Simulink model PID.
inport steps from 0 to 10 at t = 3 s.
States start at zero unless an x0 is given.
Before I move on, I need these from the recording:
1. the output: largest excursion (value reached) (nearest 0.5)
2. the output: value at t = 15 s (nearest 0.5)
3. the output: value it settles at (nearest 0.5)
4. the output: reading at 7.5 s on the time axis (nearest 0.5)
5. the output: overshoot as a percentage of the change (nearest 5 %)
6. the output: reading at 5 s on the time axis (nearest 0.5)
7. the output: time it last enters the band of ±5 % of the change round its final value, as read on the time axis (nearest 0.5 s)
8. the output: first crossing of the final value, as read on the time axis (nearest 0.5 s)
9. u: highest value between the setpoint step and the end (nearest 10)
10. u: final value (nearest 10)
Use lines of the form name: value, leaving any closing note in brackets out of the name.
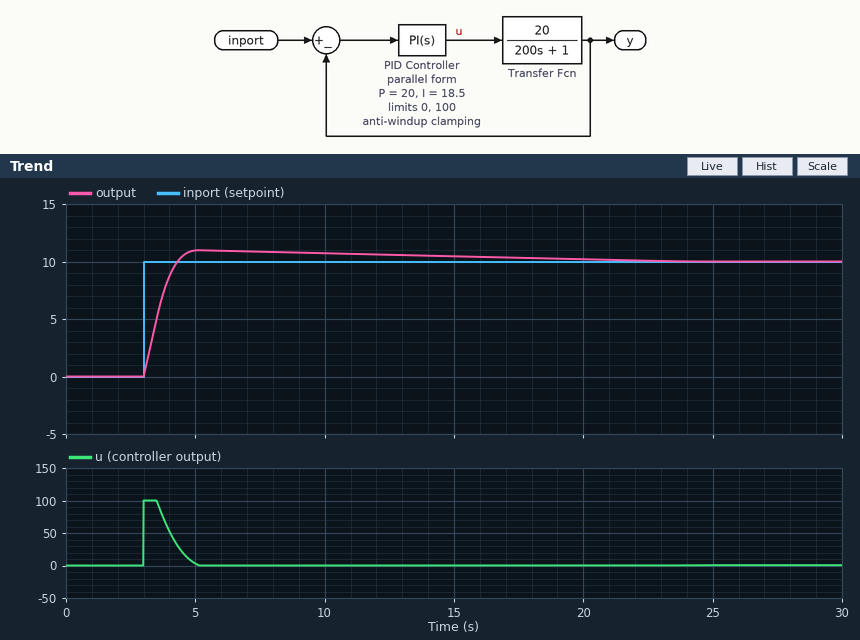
the output: largest excursion (value reached): 11.0
the output: value at t = 15 s: 10.5
the output: value it settles at: 10.0
the output: reading at 7.5 s on the time axis: 11.0
the output: overshoot as a percentage of the change: 10 %
the output: reading at 5 s on the time axis: 11.0
the output: time it last enters the band of ±5 % of the change round its final value, as read on the time axis: 14.0 s
the output: first crossing of the final value, as read on the time axis: 4.5 s
u: highest value between the setpoint step and the end: 100
u: final value: 0
